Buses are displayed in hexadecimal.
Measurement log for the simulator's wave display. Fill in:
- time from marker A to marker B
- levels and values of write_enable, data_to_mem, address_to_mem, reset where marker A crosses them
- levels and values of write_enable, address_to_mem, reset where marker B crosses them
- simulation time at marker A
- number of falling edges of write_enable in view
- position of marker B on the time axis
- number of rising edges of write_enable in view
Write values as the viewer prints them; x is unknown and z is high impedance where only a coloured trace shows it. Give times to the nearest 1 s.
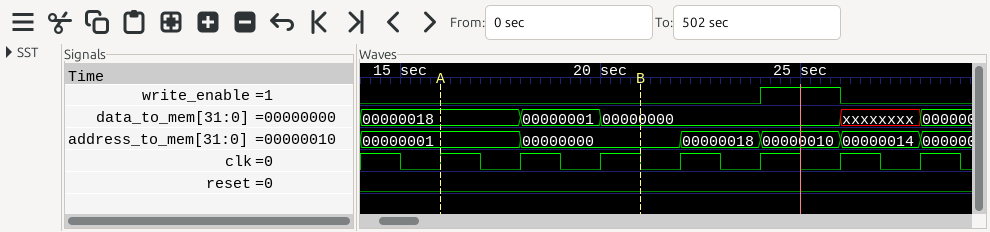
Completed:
5 s
write_enable=0, data_to_mem=00000018, address_to_mem=00000001, reset=0
write_enable=0, address_to_mem=00000000, reset=0
16 s
1
21 s
1
